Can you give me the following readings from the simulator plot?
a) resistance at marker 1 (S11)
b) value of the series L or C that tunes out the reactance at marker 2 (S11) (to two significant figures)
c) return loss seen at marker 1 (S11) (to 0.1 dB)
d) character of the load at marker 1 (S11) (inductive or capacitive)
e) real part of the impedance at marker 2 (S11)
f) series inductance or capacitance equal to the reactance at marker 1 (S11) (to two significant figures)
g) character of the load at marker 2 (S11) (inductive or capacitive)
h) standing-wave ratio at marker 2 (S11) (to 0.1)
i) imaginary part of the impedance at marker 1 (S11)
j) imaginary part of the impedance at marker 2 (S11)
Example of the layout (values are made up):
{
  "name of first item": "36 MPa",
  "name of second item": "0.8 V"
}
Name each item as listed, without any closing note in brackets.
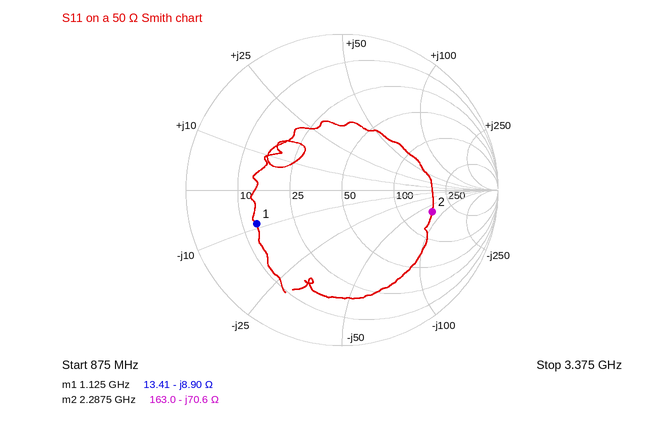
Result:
{
  "resistance at marker 1": "13.41 Ω",
  "value of the series L or C that tunes out the reactance at marker 2 (S11)": "4.9 nH",
  "return loss seen at marker 1 (S11)": "4.6 dB",
  "character of the load at marker 1 (S11)": "capacitive",
  "real part of the impedance at marker 2": "163.0 Ω",
  "series inductance or capacitance equal to the reactance at marker 1 (S11)": "16 pF",
  "character of the load at marker 2 (S11)": "capacitive",
  "standing-wave ratio at marker 2 (S11)": "3.9",
  "imaginary part of the impedance at marker 1": "-8.90 Ω",
  "imaginary part of the impedance at marker 2": "-70.6 Ω"
}
